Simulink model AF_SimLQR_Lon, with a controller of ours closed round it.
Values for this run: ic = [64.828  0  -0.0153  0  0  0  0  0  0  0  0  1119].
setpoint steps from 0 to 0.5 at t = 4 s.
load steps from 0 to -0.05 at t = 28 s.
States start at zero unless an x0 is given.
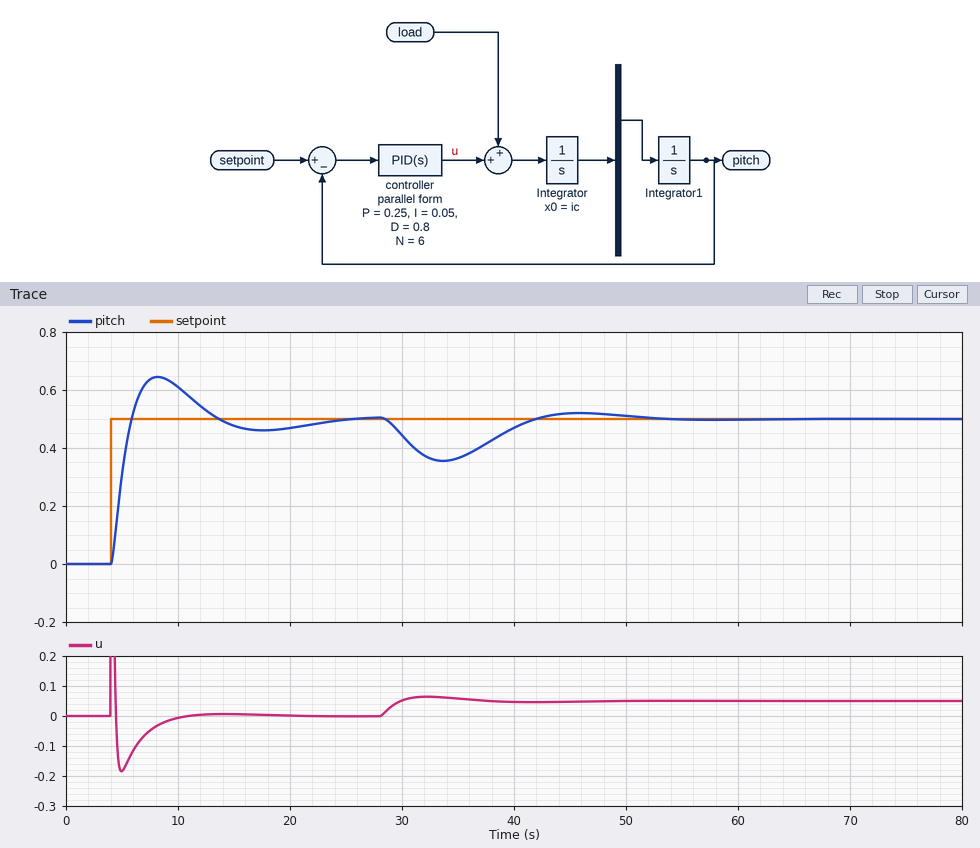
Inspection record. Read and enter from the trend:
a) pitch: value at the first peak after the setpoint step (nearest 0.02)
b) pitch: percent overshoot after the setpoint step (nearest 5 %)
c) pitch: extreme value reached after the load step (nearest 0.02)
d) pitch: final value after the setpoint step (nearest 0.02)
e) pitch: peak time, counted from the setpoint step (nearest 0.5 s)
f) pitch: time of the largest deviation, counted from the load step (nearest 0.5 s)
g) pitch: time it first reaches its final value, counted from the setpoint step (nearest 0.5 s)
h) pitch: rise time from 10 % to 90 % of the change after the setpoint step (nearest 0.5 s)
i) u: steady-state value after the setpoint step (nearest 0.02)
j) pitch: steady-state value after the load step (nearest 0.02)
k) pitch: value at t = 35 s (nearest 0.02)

0.64
30 %
0.36
0.50
4.0 s
5.5 s
2.0 s
1.5 s
0.00
0.50
0.36
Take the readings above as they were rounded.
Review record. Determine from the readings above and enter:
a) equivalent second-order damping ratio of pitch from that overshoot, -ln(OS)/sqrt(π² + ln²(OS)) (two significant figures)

0.36
